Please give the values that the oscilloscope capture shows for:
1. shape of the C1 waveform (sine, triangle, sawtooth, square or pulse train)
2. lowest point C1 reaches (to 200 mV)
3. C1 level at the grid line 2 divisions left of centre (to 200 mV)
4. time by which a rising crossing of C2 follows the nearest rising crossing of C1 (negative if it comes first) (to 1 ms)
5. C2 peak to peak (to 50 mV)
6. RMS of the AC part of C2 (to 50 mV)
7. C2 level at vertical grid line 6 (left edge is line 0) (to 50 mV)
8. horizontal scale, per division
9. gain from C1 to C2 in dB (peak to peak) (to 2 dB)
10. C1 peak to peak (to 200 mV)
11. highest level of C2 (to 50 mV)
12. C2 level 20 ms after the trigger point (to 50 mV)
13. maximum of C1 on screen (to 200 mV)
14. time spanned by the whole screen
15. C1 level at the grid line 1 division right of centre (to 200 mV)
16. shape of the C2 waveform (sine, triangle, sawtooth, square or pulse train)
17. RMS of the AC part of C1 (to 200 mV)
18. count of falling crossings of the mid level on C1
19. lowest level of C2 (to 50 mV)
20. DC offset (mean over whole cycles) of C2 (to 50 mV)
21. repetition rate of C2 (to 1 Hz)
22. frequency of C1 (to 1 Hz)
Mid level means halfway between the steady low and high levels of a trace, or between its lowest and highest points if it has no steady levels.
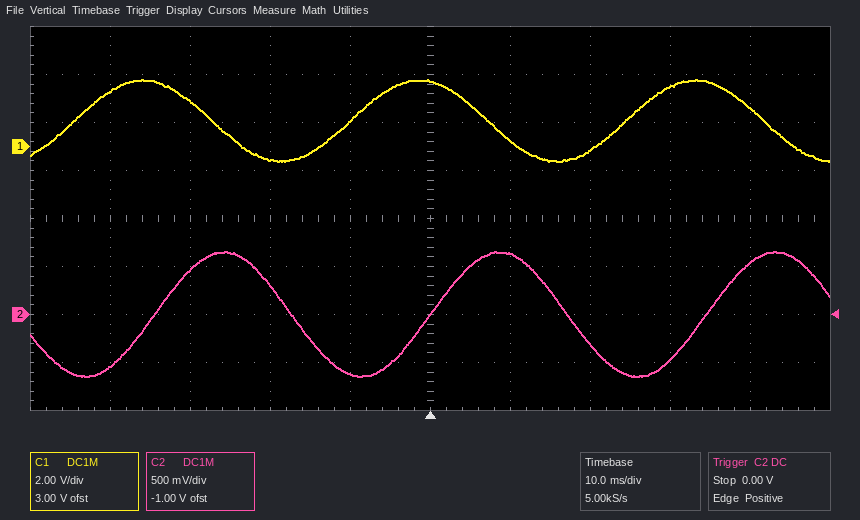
sine
-600 mV
-600 mV
+10 ms
1.30 V
450 mV
650 mV
10 ms
-8 dB
3.4 V
650 mV
-300 mV
2.8 V
100 ms
200 mV
sine
1.2 V
3
-650 mV
0 mV
29 Hz
29 Hz
